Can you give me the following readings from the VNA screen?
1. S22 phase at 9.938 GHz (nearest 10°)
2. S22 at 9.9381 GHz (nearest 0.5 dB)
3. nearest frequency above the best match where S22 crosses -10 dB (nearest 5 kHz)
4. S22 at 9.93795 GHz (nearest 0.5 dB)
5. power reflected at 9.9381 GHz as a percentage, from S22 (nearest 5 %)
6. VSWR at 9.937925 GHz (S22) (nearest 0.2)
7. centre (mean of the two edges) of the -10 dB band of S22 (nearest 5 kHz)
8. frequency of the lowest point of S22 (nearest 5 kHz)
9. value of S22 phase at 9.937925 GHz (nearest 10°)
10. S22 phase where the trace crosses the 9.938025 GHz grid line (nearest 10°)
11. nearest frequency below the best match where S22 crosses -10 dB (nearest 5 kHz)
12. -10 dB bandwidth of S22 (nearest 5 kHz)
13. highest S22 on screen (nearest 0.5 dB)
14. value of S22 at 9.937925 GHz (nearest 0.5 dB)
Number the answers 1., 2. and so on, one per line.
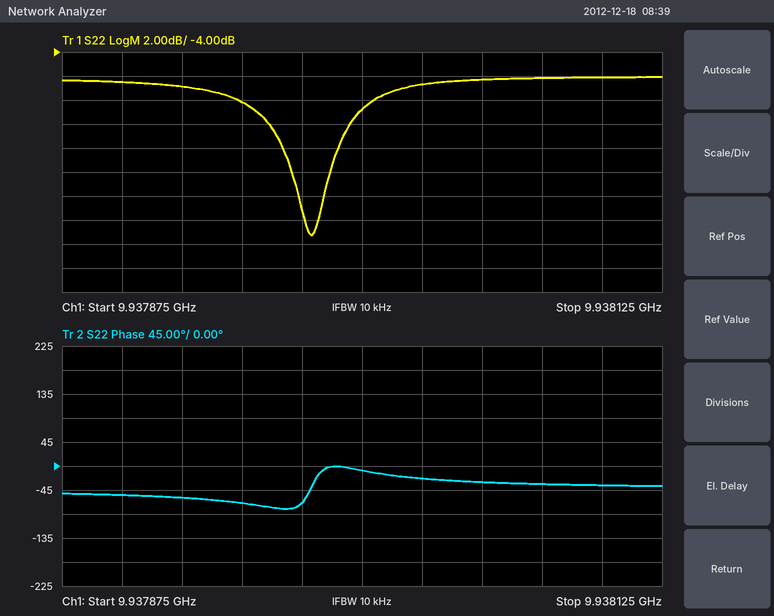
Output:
1. -10°
2. -6.0 dB
3. 9.937995 GHz
4. -8.0 dB
5. 25 %
6. 2.6
7. 9.937980 GHz
8. 9.937980 GHz
9. -60°
10. -20°
11. 9.937960 GHz
12. 35 kHz
13. -6.0 dB
14. -7.0 dB
